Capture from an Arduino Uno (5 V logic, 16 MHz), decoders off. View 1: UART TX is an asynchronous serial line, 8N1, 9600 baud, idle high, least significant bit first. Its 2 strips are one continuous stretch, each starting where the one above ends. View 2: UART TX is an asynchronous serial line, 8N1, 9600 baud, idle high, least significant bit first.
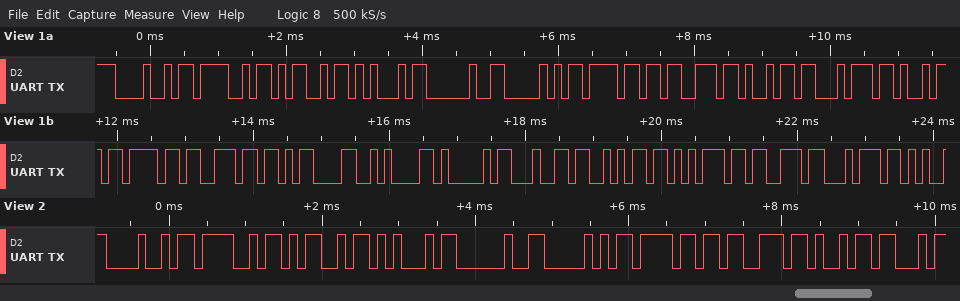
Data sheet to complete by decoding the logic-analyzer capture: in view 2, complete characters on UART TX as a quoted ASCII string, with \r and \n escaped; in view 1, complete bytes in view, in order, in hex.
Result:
"HOME Posi"
0x48 0x4F 0x4D 0x45 0x20 0x50 0x6F 0x73 0x69 0x74 0x69 0x6F 0x6E 0x0D 0x0A 0x41 0x64 0x6A 0x75 0x73 0x74
